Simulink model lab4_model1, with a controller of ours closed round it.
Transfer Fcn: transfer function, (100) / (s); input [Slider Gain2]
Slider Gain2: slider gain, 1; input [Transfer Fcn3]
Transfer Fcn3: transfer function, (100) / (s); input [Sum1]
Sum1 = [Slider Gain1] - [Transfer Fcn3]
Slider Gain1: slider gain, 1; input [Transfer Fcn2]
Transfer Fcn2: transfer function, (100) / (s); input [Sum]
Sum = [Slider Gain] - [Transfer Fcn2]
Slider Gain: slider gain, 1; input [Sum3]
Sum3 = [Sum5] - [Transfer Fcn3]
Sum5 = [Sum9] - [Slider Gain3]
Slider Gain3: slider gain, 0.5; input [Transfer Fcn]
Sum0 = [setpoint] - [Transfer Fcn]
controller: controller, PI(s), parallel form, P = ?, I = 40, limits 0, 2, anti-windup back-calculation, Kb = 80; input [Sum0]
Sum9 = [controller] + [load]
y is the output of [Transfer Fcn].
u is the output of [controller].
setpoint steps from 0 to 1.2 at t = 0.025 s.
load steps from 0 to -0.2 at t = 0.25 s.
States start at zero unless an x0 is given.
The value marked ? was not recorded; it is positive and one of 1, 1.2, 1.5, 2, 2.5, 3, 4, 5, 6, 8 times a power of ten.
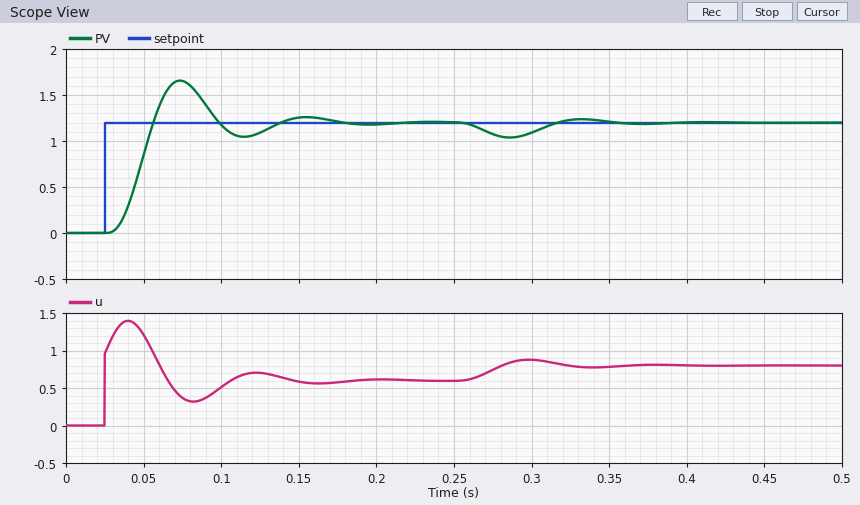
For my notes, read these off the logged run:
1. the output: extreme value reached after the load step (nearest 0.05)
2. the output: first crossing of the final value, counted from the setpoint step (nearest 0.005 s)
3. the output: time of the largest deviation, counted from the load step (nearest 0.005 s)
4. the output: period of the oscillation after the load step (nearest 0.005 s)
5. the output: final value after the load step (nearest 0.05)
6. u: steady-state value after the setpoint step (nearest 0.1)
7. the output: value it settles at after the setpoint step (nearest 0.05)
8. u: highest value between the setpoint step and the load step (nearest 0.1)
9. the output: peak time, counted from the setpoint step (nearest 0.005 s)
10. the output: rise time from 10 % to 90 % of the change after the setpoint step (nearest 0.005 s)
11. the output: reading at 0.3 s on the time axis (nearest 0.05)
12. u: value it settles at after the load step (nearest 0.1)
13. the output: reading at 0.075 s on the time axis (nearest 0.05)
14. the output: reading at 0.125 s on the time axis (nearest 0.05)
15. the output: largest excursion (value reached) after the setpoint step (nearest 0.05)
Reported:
1.05
0.030 s
0.035 s
0.085 s
1.20
0.6
1.20
1.4
0.050 s
0.020 s
1.10
0.8
1.65
1.10
1.65
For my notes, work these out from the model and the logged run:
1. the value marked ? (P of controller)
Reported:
0.8
